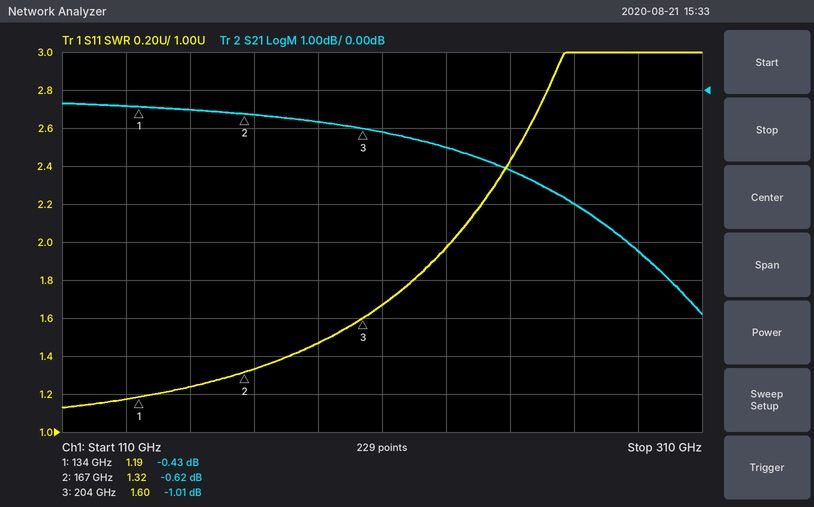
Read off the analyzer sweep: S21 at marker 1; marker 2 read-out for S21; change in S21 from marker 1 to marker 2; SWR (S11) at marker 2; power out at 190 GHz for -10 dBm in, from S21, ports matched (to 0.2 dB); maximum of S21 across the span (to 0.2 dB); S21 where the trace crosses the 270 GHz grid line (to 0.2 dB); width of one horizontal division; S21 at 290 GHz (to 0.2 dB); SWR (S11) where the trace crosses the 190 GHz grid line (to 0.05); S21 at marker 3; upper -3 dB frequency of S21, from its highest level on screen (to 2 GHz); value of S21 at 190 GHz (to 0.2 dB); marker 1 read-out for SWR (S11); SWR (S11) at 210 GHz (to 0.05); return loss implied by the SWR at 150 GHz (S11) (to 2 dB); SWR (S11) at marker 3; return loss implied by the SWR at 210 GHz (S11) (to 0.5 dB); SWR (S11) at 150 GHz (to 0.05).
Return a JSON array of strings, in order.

["-0.43 dB", "-0.62 dB", "-0.19 dB", "1.32", "-10.8 dBm", "-0.4 dB", "-3.0 dB", "20 GHz", "-4.2 dB", "1.45", "-1.01 dB", "276 GHz", "-0.8 dB", "1.19", "1.65", "20 dB", "1.60", "12.0 dB", "1.25"]
